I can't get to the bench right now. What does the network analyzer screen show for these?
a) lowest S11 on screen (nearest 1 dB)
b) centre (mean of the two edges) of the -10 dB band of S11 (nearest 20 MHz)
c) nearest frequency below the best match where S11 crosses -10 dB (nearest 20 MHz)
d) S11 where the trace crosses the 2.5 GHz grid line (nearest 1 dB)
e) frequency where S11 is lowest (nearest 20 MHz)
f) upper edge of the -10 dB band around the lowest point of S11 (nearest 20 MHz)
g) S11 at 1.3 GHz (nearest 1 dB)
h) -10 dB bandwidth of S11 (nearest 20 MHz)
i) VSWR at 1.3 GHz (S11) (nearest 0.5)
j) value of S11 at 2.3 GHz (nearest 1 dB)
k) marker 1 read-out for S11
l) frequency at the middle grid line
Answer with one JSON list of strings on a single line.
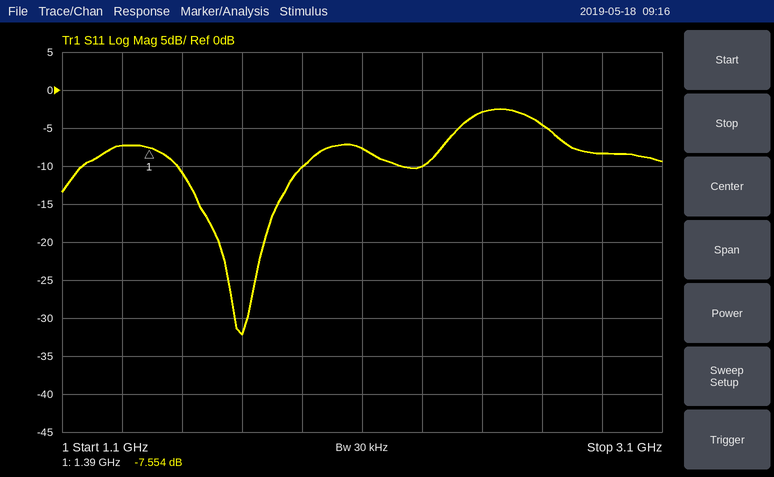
["-32 dB", "1.70 GHz", "1.48 GHz", "-3 dB", "1.70 GHz", "1.90 GHz", "-7 dB", "420 MHz", "2.5", "-10 dB", "-7.554 dB", "2.1 GHz"]
